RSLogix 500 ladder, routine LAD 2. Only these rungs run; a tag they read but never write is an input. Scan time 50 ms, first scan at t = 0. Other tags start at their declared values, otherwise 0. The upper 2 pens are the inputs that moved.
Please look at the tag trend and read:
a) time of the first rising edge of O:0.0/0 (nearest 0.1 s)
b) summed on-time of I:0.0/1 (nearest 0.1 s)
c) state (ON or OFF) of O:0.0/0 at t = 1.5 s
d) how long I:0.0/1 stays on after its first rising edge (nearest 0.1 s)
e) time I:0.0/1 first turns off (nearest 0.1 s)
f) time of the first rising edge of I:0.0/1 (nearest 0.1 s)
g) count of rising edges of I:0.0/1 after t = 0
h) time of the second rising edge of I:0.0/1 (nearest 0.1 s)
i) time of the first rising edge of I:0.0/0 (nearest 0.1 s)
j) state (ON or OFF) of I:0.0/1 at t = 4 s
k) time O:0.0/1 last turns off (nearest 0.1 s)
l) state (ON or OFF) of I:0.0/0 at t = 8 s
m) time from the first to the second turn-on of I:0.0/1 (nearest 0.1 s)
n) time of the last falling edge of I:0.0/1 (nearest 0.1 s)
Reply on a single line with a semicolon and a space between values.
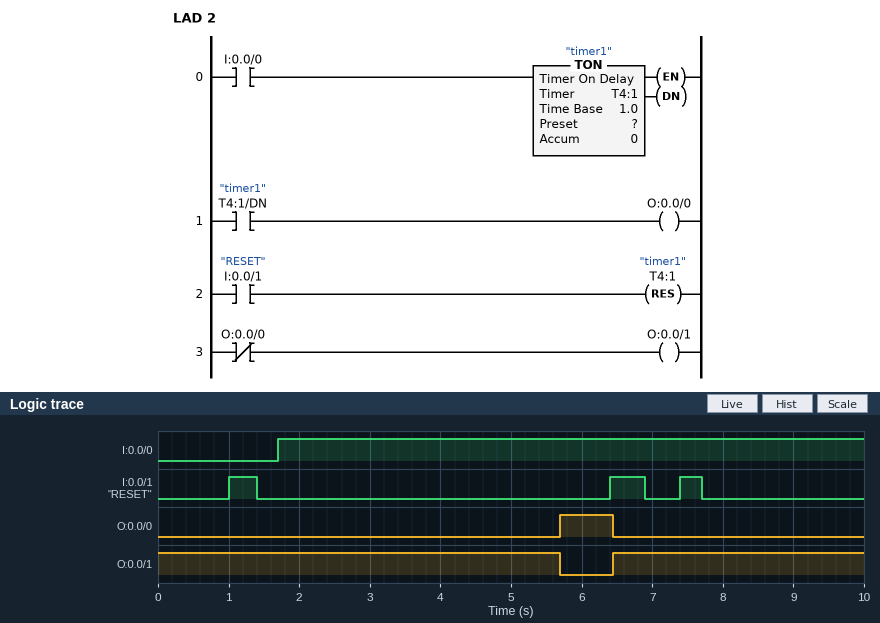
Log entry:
5.7 s; 1.2 s; OFF; 0.4 s; 1.4 s; 1.0 s; 3; 6.4 s; 1.7 s; OFF; 5.7 s; ON; 5.4 s; 7.7 s
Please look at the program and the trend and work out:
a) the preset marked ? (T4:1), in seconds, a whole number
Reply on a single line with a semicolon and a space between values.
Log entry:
4 s
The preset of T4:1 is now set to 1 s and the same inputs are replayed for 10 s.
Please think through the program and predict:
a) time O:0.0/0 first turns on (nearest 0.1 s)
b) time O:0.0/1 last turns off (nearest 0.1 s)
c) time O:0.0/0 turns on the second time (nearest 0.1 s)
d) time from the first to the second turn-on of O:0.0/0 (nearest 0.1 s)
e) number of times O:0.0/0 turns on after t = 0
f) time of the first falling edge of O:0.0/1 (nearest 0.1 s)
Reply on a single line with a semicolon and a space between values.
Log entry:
2.7 s; 8.7 s; 8.7 s; 6.0 s; 2; 2.7 s
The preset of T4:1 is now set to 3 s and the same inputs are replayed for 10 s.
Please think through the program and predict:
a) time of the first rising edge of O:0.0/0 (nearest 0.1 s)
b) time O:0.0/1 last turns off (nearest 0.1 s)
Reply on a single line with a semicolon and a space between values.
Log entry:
4.7 s; 4.7 s
